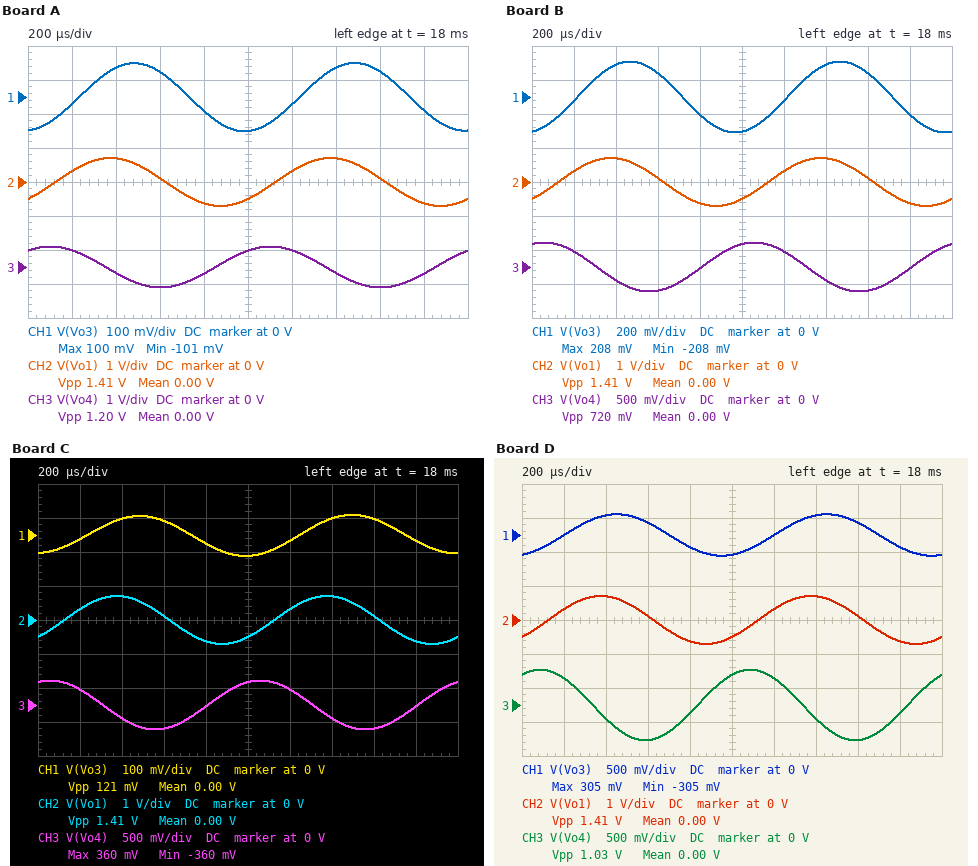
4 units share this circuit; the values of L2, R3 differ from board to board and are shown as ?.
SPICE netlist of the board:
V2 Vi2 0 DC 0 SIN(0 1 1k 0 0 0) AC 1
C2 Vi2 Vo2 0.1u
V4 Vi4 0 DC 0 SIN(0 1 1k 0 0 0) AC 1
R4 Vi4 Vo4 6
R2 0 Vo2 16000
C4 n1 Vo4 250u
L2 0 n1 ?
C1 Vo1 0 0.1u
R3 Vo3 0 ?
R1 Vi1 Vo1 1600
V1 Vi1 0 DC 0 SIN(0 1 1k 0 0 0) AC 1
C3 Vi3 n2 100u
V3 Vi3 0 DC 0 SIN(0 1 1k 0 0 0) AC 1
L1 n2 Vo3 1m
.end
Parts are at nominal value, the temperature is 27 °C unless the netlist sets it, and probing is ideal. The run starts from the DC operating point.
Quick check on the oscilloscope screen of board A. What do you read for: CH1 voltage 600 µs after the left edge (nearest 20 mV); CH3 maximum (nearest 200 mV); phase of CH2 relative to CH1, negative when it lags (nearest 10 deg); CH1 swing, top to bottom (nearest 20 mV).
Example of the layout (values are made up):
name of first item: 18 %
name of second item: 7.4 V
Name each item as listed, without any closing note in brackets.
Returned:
CH1 voltage 600 µs after the left edge: 80 mV
CH3 maximum: 600 mV
phase of CH2 relative to CH1, negative when it lags: 40 deg
CH1 swing, top to bottom: 200 mV
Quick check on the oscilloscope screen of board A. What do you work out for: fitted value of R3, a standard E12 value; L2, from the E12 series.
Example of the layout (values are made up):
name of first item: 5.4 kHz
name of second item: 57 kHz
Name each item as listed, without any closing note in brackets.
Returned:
fitted value of R3, a standard E12 value: 0.47 Ω
L2, from the E12 series: 820 µH
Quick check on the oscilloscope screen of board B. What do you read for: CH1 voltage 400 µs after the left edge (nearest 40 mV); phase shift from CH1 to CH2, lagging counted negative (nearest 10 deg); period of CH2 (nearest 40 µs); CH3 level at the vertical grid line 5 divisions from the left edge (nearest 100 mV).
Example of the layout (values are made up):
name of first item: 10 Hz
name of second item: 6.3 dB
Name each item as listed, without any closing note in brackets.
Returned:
CH1 voltage 400 µs after the left edge: 200 mV
phase shift from CH1 to CH2, lagging counted negative: 30 deg
period of CH2: 1.00 ms
CH3 level at the vertical grid line 5 divisions from the left edge: 300 mV
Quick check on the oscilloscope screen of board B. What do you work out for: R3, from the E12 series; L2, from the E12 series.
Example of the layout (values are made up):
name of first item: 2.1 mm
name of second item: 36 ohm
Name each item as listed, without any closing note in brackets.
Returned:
R3, from the E12 series: 1 Ω
L2, from the E12 series: 470 µH
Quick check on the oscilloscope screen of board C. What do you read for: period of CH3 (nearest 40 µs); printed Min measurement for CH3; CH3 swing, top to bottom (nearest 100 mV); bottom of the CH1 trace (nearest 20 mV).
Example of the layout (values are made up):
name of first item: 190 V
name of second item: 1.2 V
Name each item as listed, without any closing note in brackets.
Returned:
period of CH3: 1.00 ms
printed Min measurement for CH3: -360 mV
CH3 swing, top to bottom: 700 mV
bottom of the CH1 trace: -60 mV
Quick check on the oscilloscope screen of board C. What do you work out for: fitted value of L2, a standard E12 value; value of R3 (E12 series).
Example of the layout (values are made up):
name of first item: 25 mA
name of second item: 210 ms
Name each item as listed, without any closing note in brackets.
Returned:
fitted value of L2, a standard E12 value: 470 µH
value of R3: 0.27 Ω
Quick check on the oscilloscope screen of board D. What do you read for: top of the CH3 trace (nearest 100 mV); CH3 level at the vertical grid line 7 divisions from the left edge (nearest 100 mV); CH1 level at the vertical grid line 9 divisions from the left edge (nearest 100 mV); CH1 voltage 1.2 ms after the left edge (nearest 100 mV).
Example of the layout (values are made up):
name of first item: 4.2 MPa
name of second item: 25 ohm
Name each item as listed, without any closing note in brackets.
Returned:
top of the CH3 trace: 500 mV
CH3 level at the vertical grid line 7 divisions from the left edge: -200 mV
CH1 level at the vertical grid line 9 divisions from the left edge: -200 mV
CH1 voltage 1.2 ms after the left edge: 0 V
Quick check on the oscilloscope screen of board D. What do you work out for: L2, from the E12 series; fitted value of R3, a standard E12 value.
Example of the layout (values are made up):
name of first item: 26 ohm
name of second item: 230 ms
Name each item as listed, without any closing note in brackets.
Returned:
L2, from the E12 series: 680 µH
fitted value of R3, a standard E12 value: 1.5 Ω
